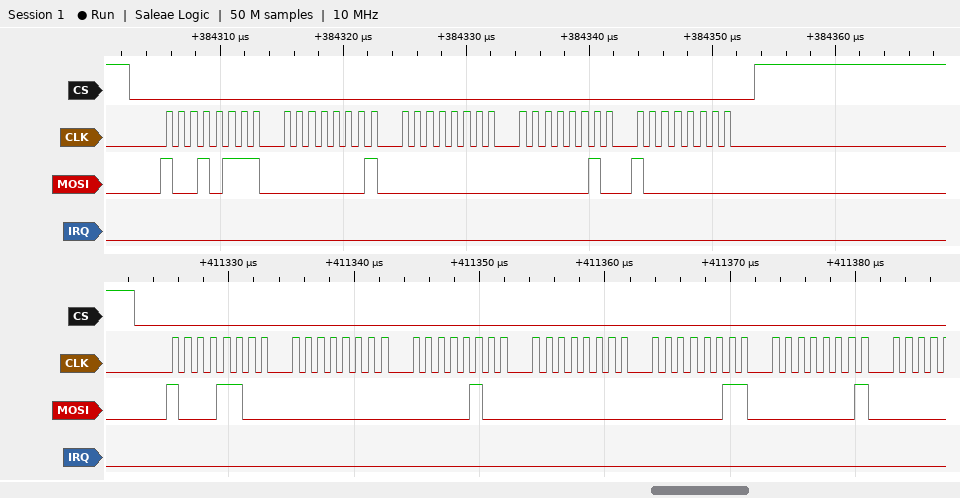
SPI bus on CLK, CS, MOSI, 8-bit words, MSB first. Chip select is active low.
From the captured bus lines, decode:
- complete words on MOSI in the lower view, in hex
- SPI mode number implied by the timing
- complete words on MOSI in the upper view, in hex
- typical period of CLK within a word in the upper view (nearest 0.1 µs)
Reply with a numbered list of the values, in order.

1. 8C, 00, 04, 00, 03, 01
2. 0
3. 97, 01, 00, 02, 80
4. 1 µs
